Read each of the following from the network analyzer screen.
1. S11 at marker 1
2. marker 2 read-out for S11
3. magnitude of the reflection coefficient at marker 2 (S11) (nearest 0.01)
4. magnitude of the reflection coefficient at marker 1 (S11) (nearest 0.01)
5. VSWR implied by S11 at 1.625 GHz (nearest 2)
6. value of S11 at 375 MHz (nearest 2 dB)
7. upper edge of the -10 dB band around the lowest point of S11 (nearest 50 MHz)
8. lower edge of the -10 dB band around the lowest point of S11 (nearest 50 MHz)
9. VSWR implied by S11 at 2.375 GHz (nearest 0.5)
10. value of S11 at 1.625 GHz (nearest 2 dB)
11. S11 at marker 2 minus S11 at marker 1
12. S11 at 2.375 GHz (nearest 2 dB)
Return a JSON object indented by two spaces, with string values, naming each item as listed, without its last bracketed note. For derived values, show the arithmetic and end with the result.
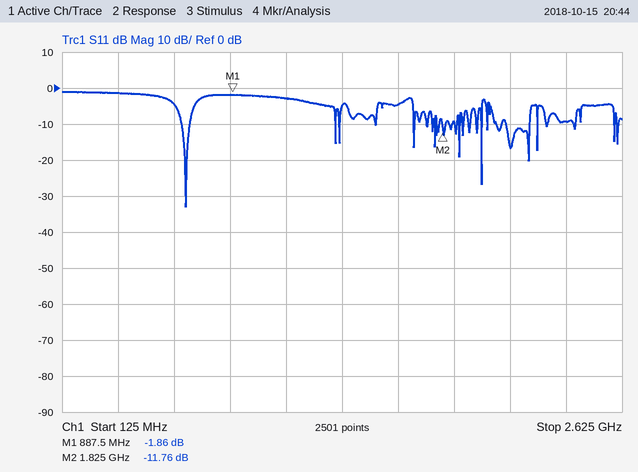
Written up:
{
  "S11 at marker 1": "-1.86 dB",
  "marker 2 read-out for S11": "-11.76 dB",
  "magnitude of the reflection coefficient at marker 2 (S11)": "10^(-11.76/20) ≈ 0.26",
  "magnitude of the reflection coefficient at marker 1 (S11)": "10^(-1.86/20) ≈ 0.81",
  "VSWR implied by S11 at 1.625 GHz": "|Γ| = 10^(-4/20) = 0.6310; VSWR = (1 + 0.6310)/(1 − 0.6310) ≈ 4",
  "value of S11 at 375 MHz": "-2 dB",
  "upper edge of the -10 dB band around the lowest point of S11": "700 MHz",
  "lower edge of the -10 dB band around the lowest point of S11": "650 MHz",
  "VSWR implied by S11 at 2.375 GHz": "|Γ| = 10^(-10/20) = 0.3162; VSWR = (1 + 0.3162)/(1 − 0.3162) ≈ 1.92, so 2.0 to the nearest 0.5",
  "value of S11 at 1.625 GHz": "-4 dB",
  "S11 at marker 2 minus S11 at marker 1": "-11.76 − (-1.86) = -9.90 dB",
  "S11 at 2.375 GHz": "-10 dB"
}
